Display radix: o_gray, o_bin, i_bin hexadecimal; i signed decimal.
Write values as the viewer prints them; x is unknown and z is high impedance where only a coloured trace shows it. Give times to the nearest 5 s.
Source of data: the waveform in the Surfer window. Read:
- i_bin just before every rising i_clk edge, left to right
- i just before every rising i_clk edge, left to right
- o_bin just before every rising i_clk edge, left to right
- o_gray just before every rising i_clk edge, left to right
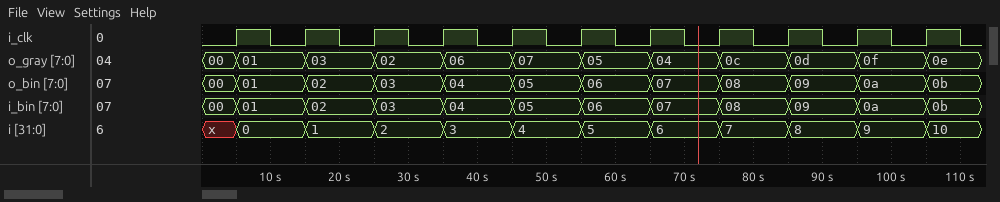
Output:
00, 01, 02, 03, 04, 05, 06, 07, 08, 09, 0a
x, 0, 1, 2, 3, 4, 5, 6, 7, 8, 9
00, 01, 02, 03, 04, 05, 06, 07, 08, 09, 0a
00, 01, 03, 02, 06, 07, 05, 04, 0c, 0d, 0f
